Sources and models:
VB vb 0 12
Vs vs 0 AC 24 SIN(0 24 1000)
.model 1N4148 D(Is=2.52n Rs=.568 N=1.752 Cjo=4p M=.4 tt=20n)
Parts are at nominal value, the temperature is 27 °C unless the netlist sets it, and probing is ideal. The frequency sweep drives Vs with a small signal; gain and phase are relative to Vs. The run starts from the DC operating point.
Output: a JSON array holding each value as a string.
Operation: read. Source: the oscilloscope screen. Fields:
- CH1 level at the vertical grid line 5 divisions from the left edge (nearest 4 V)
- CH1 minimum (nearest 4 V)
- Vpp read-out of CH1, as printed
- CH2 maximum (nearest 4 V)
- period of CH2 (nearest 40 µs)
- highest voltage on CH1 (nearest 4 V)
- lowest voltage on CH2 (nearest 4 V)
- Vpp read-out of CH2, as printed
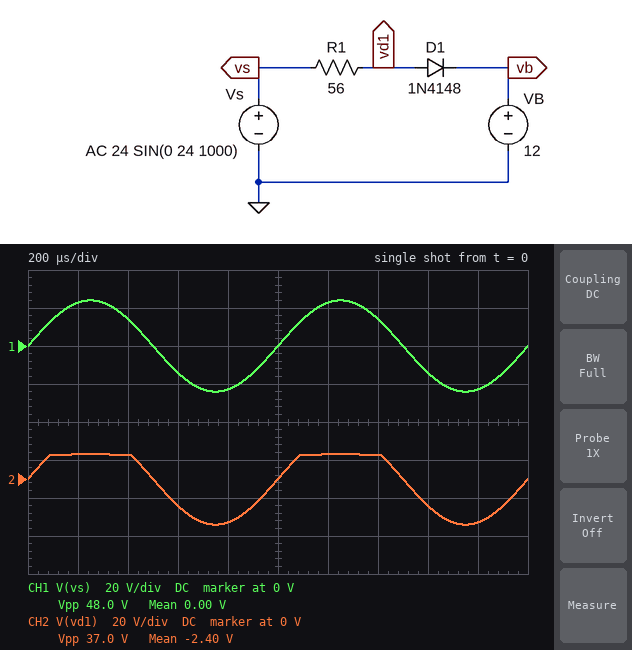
["0 V", "-24 V", "48.0 V", "12 V", "1.00 ms", "24 V", "-24 V", "37.0 V"]
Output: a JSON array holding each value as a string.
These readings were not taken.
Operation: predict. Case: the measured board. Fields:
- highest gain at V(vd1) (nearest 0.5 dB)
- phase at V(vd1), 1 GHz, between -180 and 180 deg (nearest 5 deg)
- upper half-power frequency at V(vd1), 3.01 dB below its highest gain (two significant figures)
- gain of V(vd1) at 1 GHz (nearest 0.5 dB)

["0 dB", "-25 deg", "2.0 GHz", "-1.0 dB"]
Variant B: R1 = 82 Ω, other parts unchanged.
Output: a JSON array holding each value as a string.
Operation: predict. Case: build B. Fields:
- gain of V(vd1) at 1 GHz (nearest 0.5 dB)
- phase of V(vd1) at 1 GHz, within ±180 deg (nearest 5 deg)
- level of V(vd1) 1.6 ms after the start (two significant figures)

["-2.0 dB", "-35 deg", "-14 V"]
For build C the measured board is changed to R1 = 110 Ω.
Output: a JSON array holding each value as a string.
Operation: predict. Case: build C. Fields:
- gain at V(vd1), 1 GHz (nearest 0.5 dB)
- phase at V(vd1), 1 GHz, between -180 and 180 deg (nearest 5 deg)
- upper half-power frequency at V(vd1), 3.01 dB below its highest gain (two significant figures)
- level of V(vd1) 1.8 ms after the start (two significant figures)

["-3.0 dB", "-45 deg", "1.0 GHz", "-23 V"]
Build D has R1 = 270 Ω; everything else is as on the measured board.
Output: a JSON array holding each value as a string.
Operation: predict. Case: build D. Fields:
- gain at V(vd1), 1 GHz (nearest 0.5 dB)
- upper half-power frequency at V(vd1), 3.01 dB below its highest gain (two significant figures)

["-8.5 dB", "410 MHz"]
